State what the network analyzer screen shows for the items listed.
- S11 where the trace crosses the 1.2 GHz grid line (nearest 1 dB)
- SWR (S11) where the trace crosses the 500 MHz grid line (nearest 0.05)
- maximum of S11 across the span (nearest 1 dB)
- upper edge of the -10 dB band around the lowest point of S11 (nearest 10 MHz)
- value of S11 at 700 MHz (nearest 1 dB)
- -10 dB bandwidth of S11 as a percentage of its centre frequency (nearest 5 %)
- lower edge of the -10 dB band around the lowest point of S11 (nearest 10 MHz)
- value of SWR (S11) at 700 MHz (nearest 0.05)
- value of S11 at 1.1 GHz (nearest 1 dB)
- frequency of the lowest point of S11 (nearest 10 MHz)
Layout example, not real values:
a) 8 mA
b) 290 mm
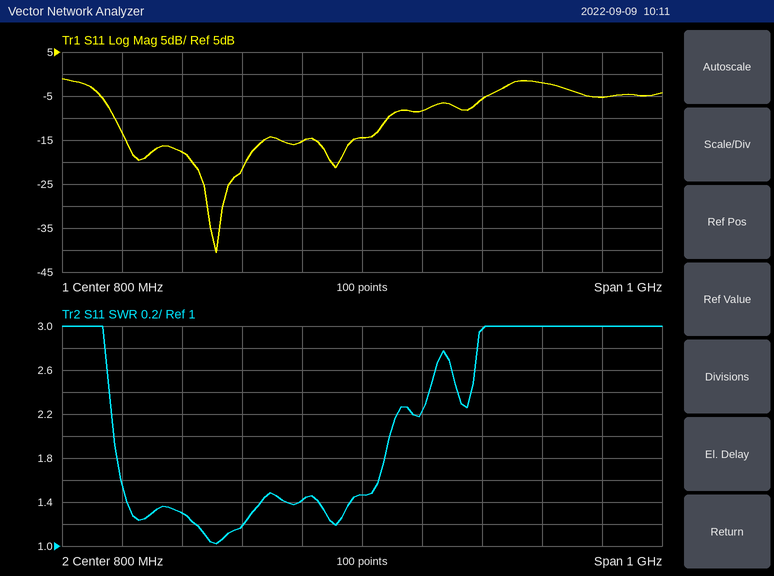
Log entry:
a) -5 dB
b) 1.30
c) -1 dB
d) 840 MHz
e) -15 dB
f) 75 %
g) 390 MHz
h) 1.40
i) -2 dB
j) 560 MHz
